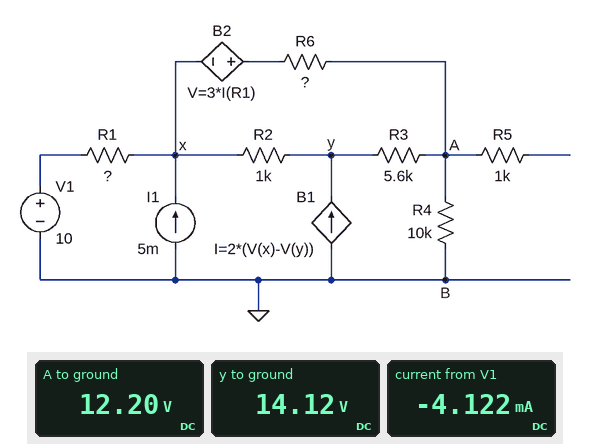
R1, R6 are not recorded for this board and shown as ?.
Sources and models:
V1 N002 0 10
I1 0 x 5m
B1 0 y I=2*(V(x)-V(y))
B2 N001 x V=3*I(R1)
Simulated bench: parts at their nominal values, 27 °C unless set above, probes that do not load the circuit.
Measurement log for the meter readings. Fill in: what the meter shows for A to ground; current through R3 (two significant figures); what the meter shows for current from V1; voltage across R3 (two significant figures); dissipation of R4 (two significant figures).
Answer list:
12.20 V
340 µA
-4.122 mA
1.9 V
15 mW
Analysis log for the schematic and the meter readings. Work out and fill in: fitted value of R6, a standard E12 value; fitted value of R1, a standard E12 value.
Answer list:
2.2 kΩ
1 kΩ
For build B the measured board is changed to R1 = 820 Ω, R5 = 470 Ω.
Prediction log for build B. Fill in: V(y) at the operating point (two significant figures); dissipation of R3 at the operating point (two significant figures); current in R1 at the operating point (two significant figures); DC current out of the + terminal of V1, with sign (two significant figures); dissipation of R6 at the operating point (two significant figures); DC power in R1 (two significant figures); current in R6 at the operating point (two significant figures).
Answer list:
13 V
590 µW
4.2 mA
-4.2 mA
1.5 mW
14 mW
830 µA
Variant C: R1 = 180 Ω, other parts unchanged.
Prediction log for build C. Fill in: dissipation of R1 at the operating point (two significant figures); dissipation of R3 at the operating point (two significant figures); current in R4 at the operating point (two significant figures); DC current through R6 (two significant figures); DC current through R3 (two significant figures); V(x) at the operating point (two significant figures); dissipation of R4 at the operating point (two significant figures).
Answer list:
3.4 mW
380 µW
930 µA
670 µA
260 µA
11 V
8.7 mW
